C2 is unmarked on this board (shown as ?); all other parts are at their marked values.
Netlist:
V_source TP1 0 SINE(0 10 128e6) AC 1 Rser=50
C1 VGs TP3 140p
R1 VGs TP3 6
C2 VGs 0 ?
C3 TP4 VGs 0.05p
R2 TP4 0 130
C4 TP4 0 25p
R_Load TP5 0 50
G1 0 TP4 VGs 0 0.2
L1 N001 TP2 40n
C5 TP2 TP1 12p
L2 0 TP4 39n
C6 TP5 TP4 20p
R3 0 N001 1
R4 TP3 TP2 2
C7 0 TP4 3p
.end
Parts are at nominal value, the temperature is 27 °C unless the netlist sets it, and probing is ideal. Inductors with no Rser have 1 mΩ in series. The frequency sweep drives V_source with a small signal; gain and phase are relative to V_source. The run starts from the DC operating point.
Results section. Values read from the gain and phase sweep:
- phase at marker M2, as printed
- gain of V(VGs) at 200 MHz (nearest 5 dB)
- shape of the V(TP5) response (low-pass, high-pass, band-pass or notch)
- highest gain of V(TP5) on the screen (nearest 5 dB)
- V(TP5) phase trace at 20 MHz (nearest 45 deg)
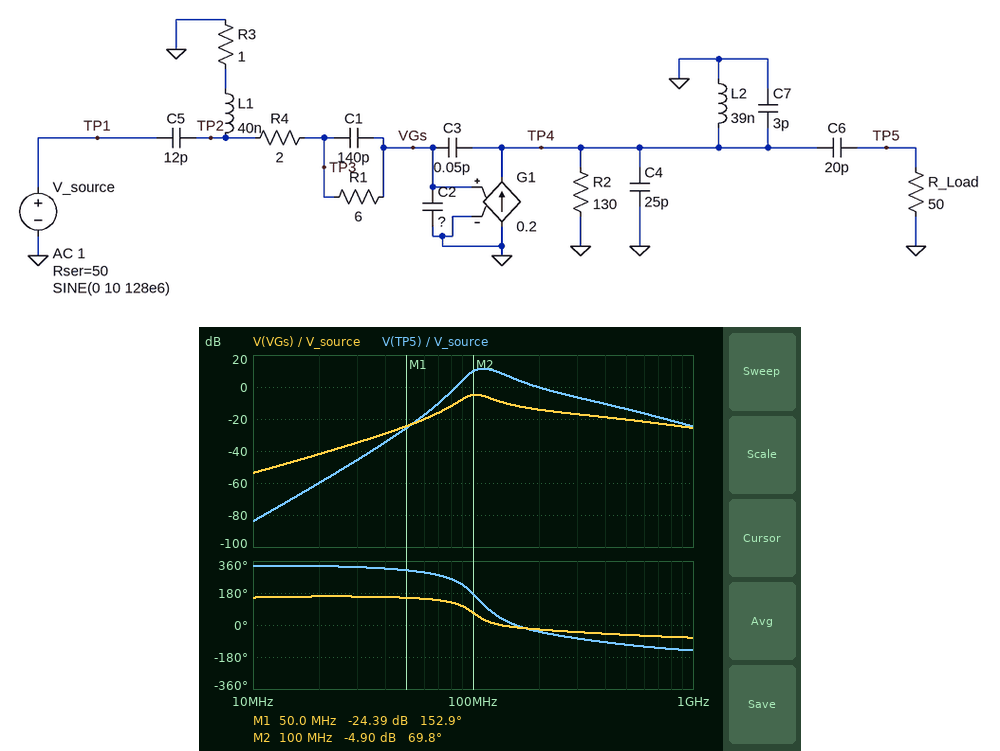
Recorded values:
69.8 deg
-15 dB
band-pass
10 dB
315 deg
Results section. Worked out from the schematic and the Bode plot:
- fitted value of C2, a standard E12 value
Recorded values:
56 pF
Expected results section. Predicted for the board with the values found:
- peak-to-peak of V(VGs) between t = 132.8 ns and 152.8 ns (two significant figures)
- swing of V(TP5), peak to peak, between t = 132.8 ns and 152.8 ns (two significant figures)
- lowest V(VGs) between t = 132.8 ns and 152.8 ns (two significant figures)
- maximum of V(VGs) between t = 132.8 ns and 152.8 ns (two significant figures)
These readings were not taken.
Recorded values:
7.6 V
61 V
-3.8 V
3.8 V
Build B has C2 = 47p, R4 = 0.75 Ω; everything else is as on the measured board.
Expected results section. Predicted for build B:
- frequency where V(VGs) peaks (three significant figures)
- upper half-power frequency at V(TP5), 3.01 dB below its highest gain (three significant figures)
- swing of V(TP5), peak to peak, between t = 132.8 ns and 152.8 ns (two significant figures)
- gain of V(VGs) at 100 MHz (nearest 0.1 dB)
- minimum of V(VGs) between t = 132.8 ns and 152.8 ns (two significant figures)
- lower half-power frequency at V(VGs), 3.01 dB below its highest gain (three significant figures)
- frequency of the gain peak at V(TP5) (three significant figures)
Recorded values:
110 MHz
133 MHz
89 V
-4.1 dB
-5.5 V
97.4 MHz
114 MHz
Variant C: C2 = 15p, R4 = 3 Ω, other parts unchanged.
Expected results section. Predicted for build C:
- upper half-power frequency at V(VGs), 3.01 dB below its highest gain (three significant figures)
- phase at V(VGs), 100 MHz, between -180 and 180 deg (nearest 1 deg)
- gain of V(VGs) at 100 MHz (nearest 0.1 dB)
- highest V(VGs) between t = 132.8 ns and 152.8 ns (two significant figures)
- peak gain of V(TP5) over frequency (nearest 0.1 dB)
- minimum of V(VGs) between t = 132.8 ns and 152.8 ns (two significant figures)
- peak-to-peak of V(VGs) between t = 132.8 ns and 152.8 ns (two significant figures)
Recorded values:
199 MHz
144 deg
-11.1 dB
6.3 V
18.9 dB
-6.3 V
13 V
